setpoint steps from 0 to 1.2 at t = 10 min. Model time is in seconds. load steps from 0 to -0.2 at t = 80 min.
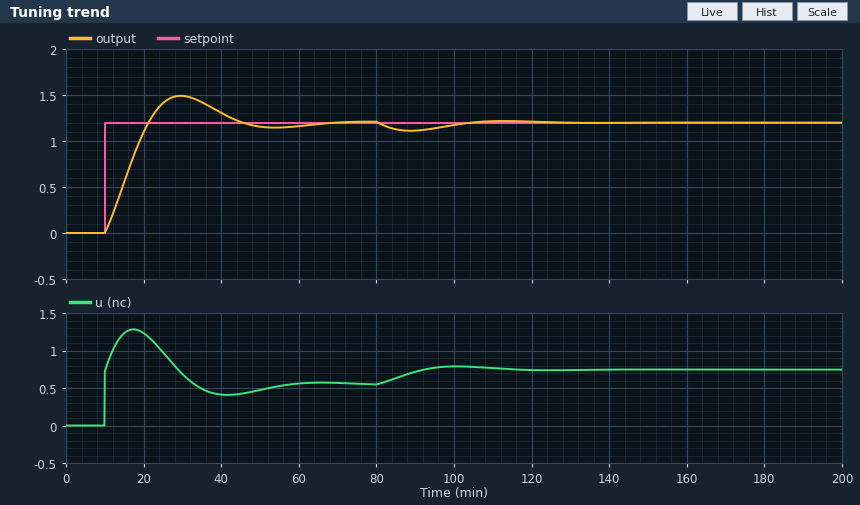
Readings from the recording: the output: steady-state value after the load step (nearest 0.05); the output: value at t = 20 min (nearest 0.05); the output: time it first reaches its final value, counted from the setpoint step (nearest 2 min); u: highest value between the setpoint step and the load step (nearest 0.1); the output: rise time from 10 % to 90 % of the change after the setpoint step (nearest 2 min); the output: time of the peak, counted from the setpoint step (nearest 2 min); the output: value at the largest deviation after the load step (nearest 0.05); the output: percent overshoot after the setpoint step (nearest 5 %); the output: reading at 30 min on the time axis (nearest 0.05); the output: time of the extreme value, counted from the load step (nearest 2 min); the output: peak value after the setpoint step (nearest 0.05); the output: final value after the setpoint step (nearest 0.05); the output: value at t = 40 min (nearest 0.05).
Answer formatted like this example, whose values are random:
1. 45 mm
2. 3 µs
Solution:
1. 1.20
2. 1.10
3. 12 min
4. 1.3
5. 8 min
6. 20 min
7. 1.10
8. 25 %
9. 1.50
10. 8 min
11. 1.50
12. 1.20
13. 1.30
